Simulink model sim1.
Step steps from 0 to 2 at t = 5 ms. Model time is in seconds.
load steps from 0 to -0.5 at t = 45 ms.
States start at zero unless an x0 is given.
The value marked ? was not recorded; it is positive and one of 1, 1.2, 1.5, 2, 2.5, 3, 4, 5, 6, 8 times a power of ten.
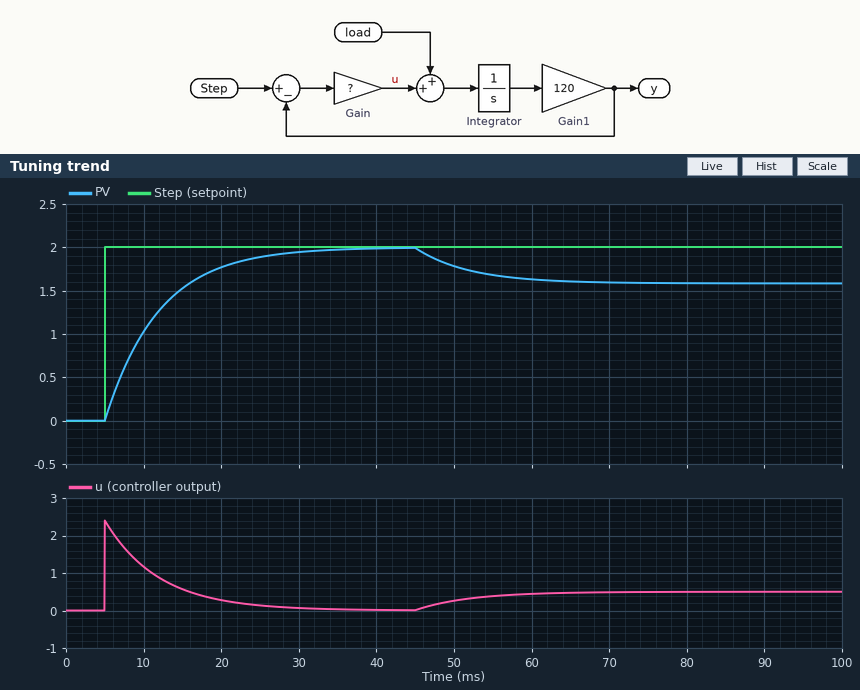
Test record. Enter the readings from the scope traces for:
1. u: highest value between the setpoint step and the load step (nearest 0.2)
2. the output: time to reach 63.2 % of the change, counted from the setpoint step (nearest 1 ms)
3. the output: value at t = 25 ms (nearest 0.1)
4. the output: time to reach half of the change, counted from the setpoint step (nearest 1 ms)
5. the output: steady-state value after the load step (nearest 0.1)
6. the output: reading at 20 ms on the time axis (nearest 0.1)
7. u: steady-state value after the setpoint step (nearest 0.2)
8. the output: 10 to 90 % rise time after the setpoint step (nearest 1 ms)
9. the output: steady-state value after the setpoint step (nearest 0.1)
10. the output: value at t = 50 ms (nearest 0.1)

2.4
7 ms
1.9
5 ms
1.6
1.8
0.0
15 ms
2.0
1.8
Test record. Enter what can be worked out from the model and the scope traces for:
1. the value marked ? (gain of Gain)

1.2
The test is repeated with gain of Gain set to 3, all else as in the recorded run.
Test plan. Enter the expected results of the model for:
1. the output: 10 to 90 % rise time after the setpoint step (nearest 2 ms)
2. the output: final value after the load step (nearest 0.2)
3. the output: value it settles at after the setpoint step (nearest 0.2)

6 ms
1.8
2.0
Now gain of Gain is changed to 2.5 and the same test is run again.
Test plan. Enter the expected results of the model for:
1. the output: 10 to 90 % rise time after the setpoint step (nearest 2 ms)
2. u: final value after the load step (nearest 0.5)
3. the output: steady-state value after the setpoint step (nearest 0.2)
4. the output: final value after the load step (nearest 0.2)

8 ms
0.5
2.0
1.8
